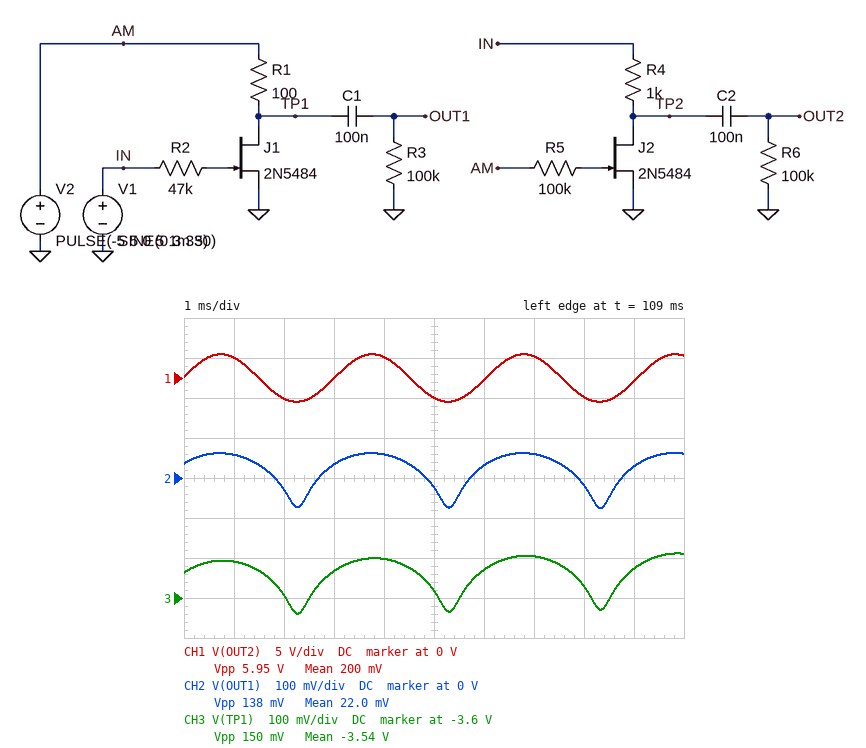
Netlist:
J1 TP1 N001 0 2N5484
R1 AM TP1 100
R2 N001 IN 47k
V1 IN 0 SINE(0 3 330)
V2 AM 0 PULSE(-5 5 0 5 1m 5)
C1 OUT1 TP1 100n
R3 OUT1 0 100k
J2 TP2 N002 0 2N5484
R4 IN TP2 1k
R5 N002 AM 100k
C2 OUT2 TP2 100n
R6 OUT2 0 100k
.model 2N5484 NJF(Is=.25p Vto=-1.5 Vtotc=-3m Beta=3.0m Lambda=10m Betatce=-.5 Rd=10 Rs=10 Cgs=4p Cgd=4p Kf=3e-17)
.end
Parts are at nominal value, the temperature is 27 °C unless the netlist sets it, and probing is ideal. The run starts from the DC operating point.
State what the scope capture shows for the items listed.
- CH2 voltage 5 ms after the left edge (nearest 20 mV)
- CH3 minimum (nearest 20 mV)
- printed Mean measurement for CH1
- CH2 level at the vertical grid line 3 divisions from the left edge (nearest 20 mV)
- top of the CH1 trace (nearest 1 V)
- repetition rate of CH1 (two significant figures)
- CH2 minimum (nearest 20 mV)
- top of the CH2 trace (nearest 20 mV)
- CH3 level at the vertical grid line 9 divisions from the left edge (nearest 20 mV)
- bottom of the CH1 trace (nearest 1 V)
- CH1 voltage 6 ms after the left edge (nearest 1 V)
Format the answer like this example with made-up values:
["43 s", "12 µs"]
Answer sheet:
["-20 mV", "-3.64 V", "200 mV", "40 mV", "3 V", "330 Hz", "-80 mV", "60 mV", "-3.52 V", "-3 V", "0 V"]
